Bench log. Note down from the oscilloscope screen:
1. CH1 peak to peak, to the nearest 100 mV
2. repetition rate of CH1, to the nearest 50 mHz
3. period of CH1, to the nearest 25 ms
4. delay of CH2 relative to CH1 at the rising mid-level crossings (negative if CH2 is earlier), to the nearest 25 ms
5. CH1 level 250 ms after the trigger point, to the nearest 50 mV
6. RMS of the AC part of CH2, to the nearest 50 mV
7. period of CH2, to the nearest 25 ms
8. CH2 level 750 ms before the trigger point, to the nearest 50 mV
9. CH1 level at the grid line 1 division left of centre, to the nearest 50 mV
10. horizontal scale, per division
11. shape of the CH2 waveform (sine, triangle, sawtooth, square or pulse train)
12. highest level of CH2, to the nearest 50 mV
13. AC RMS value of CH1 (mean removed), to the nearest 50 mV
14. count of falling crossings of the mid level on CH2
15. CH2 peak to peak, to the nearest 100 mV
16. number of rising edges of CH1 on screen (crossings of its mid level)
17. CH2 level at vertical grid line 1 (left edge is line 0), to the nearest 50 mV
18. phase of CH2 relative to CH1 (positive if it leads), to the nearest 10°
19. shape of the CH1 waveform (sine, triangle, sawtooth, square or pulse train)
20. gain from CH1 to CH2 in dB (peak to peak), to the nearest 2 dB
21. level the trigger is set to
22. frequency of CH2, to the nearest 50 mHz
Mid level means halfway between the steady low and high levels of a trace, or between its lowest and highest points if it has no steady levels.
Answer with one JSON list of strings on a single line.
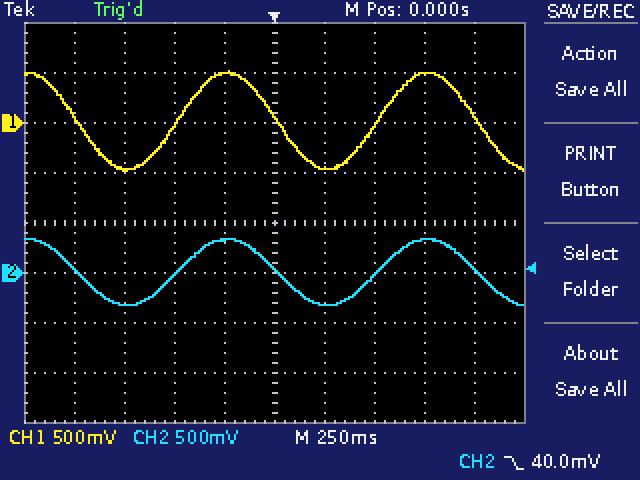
["1.00 V", "1.00 Hz", "1.000 s", "0 ms", "-450 mV", "250 mV", "1.000 s", "-300 mV", "500 mV", "250 ms", "sine", "350 mV", "350 mV", "3", "700 mV", "2", "50 mV", "0°", "sine", "-4 dB", "40.0 mV", "1.00 Hz"]
